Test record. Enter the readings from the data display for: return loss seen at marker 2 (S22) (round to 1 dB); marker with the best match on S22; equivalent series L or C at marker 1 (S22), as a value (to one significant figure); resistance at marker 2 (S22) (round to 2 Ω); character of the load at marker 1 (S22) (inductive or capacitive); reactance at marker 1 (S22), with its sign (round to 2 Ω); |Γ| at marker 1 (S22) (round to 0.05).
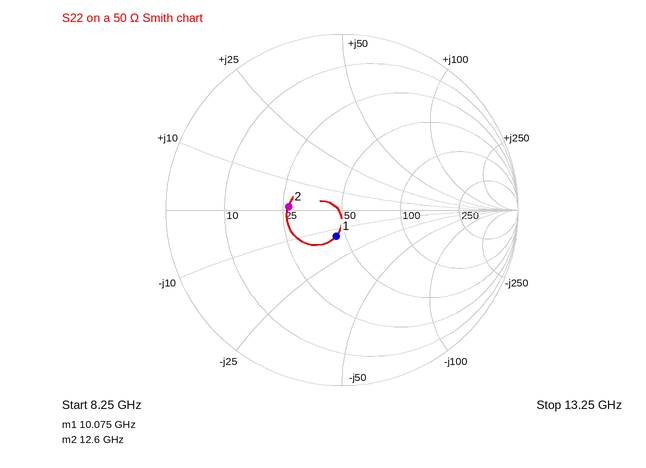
10 dB
marker 1
1 pF
26 Ω
capacitive
-14 Ω
0.15
